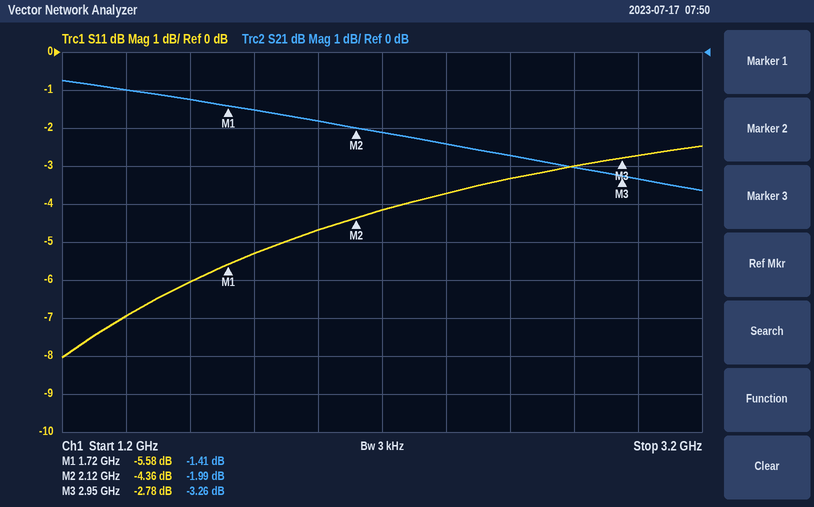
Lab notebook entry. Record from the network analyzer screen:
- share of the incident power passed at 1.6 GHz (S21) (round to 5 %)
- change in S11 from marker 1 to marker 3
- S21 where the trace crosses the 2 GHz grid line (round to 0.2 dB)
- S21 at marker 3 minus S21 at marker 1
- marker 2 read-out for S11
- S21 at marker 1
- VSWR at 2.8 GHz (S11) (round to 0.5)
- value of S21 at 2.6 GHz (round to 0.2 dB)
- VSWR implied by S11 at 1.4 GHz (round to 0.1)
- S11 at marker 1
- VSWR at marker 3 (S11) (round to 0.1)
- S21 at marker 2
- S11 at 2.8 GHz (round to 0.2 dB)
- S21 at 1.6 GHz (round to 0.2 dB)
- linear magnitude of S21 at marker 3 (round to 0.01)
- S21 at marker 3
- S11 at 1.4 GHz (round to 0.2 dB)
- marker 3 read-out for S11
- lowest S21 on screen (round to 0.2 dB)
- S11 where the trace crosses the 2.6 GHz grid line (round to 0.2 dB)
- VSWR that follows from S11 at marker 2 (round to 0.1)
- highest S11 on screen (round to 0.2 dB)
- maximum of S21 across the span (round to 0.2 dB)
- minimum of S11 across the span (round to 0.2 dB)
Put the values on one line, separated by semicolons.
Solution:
75 %; 2.80 dB; -1.8 dB; -1.85 dB; -4.36 dB; -1.41 dB; 6.0; -2.8 dB; 2.6; -5.58 dB; 6.3; -1.99 dB; -3.0 dB; -1.2 dB; 0.69; -3.26 dB; -7.0 dB; -2.78 dB; -3.6 dB; -3.4 dB; 4.1; -2.4 dB; -0.8 dB; -8.0 dB
